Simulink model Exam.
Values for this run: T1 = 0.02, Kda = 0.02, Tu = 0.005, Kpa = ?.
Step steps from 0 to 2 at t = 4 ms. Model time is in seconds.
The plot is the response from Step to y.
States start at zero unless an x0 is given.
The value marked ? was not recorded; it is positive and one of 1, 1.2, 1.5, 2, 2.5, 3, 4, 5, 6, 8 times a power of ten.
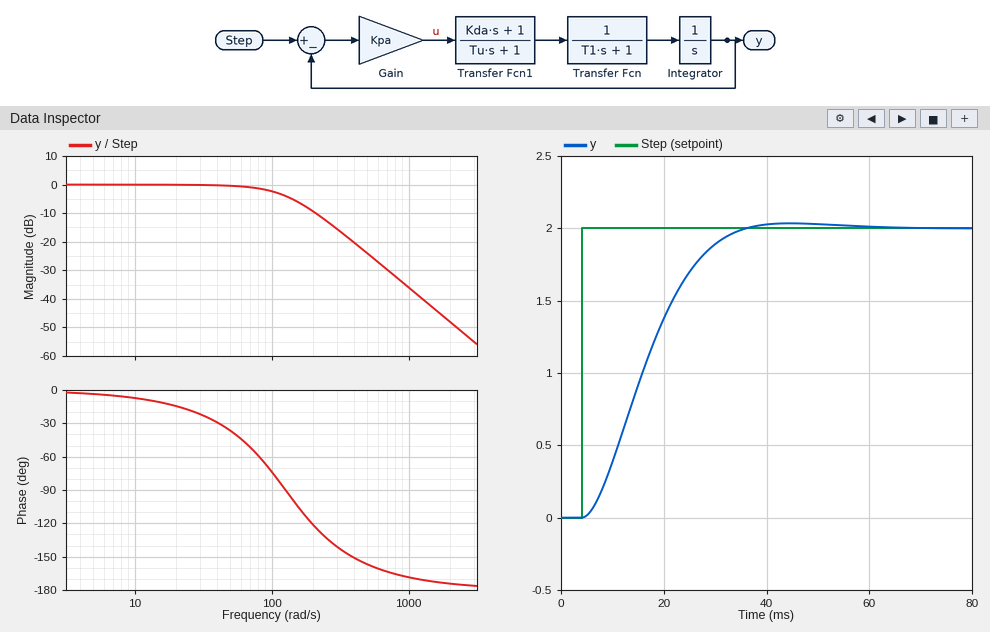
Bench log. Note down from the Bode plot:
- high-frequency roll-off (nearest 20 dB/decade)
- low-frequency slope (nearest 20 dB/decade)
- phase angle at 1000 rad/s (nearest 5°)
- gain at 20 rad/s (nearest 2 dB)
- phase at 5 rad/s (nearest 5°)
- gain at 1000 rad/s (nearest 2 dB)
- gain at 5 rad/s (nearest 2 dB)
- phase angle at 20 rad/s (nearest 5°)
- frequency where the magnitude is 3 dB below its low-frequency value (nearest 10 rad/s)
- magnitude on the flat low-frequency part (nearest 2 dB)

-40 dB/decade
0 dB/decade
-170°
0 dB
-5°
-36 dB
0 dB
-15°
110 rad/s
0 dB
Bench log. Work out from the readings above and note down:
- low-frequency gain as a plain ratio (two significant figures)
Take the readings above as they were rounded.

1.0
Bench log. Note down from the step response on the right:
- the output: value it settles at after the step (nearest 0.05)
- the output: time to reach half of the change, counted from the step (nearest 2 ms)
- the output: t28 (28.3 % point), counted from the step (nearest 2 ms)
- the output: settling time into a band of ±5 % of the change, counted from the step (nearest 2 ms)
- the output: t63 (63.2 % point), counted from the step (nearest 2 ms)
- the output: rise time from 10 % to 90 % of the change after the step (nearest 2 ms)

2.00
12 ms
8 ms
26 ms
14 ms
20 ms
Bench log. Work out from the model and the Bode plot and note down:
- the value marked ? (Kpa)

80
